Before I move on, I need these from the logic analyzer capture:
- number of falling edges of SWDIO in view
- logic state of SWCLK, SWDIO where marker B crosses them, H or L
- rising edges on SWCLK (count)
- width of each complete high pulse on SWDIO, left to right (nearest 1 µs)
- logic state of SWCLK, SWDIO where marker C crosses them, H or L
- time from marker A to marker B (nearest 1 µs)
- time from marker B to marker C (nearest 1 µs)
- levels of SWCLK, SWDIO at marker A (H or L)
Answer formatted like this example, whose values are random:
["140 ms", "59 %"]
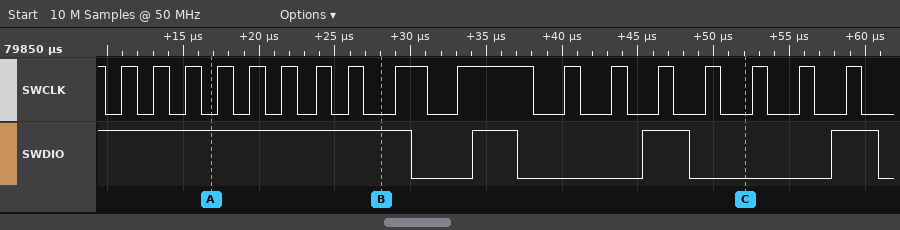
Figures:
["4", "SWCLK=L, SWDIO=H", "17", "3 µs, 3 µs, 3 µs", "SWCLK=L, SWDIO=L", "11 µs", "24 µs", "SWCLK=L, SWDIO=H"]
